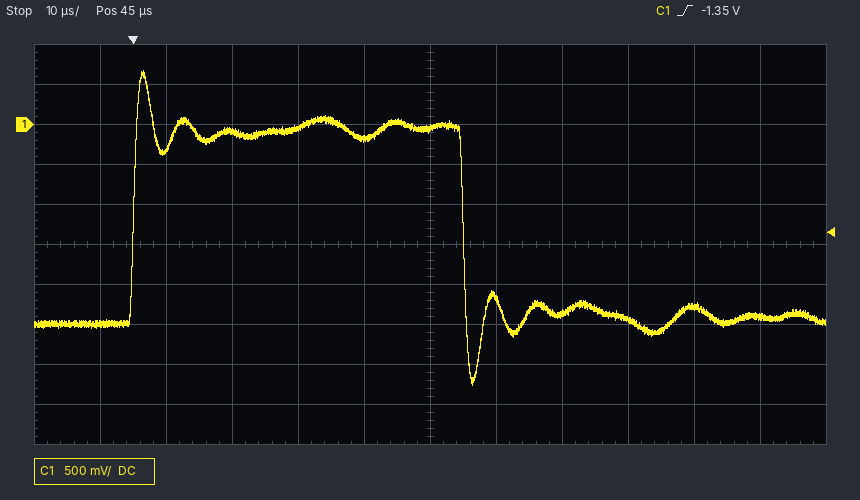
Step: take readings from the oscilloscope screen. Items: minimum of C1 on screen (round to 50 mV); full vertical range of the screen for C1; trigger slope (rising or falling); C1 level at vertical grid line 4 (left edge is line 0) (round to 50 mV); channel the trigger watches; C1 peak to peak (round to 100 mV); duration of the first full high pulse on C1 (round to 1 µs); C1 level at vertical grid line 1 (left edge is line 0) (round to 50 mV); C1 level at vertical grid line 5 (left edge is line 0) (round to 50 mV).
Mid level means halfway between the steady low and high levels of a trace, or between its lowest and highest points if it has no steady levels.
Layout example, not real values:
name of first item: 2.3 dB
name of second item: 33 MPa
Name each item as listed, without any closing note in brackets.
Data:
minimum of C1 on screen: -3.25 V
full vertical range of the screen for C1: 5 V
trigger slope: rising
C1 level at vertical grid line 4 (left edge is line 0): -50 mV
channel the trigger watches: C1
C1 peak to peak: 3.90 V
duration of the first full high pulse on C1: 50 µs
C1 level at vertical grid line 1 (left edge is line 0): -2.50 V
C1 level at vertical grid line 5 (left edge is line 0): -200 mV
